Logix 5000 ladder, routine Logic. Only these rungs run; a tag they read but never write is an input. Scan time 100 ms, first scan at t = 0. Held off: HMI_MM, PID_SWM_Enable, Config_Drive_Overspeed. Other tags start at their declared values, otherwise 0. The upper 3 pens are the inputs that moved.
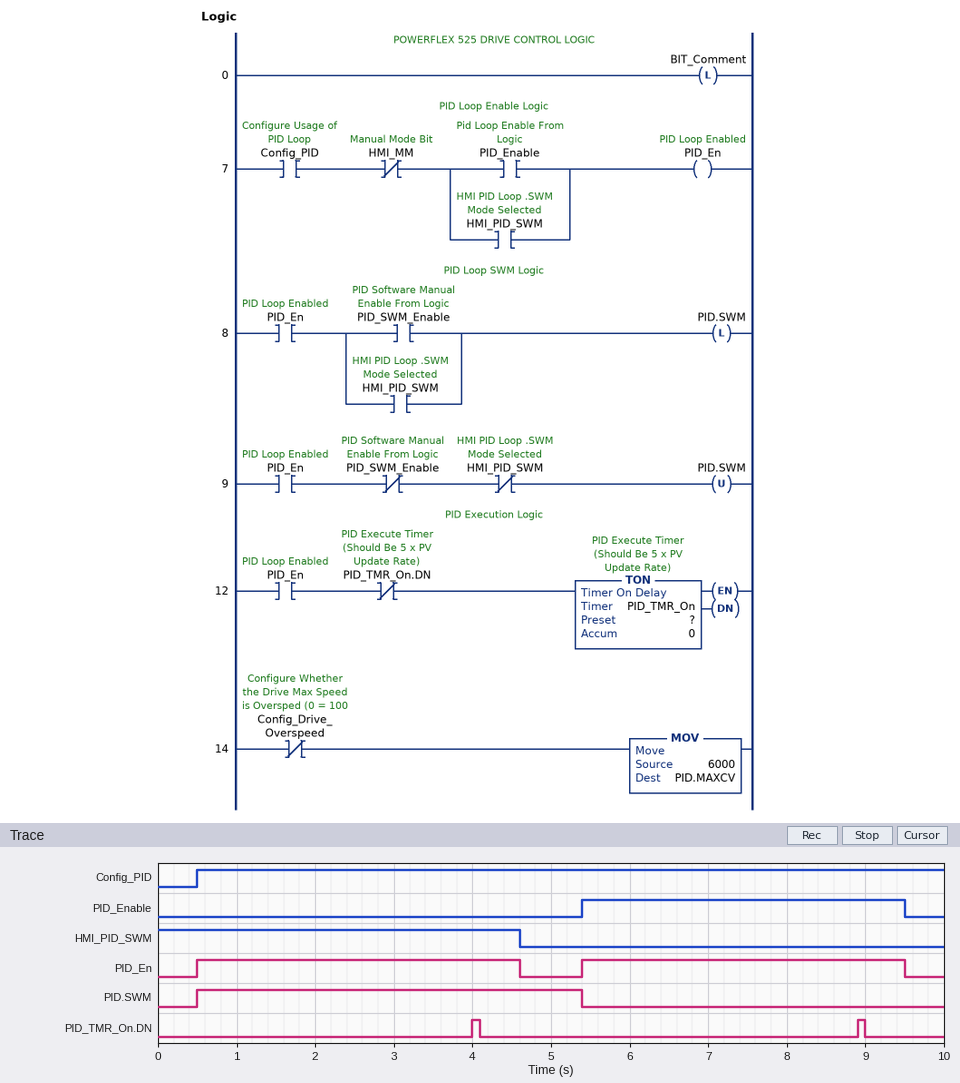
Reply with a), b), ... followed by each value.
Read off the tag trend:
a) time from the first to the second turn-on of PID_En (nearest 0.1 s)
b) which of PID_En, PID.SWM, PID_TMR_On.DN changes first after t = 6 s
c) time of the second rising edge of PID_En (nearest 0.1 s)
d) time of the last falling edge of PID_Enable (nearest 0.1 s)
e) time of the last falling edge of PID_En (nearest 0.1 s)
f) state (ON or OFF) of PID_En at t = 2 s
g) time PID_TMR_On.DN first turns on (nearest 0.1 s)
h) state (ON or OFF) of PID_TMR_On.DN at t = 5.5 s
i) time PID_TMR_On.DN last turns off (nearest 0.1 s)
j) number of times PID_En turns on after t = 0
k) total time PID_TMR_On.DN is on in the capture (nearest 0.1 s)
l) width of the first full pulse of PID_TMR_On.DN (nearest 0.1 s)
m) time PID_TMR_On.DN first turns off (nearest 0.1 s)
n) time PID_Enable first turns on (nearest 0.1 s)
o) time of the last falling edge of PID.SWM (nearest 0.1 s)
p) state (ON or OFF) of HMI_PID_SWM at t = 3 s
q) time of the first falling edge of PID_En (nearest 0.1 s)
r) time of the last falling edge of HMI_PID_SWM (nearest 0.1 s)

a) 4.9 s
b) PID_TMR_On.DN
c) 5.4 s
d) 9.5 s
e) 9.5 s
f) ON
g) 4.0 s
h) OFF
i) 9.0 s
j) 2
k) 0.2 s
l) 0.1 s
m) 4.1 s
n) 5.4 s
o) 5.4 s
p) ON
q) 4.6 s
r) 4.6 s
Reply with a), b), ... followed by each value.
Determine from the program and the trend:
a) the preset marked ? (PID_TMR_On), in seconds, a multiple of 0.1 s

a) 3.5 s
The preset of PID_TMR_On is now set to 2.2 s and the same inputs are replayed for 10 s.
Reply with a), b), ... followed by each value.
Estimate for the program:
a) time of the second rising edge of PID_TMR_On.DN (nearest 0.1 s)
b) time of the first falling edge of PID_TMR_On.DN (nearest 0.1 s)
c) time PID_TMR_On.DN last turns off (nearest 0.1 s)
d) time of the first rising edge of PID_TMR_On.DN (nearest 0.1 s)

a) 7.6 s
b) 2.8 s
c) 7.7 s
d) 2.7 s
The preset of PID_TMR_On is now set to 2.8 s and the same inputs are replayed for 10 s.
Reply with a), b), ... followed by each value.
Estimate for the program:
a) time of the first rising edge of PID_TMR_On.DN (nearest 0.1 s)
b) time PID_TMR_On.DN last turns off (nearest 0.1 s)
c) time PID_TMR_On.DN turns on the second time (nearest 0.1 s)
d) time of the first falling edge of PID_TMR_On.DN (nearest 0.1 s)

a) 3.3 s
b) 8.3 s
c) 8.2 s
d) 3.4 s
